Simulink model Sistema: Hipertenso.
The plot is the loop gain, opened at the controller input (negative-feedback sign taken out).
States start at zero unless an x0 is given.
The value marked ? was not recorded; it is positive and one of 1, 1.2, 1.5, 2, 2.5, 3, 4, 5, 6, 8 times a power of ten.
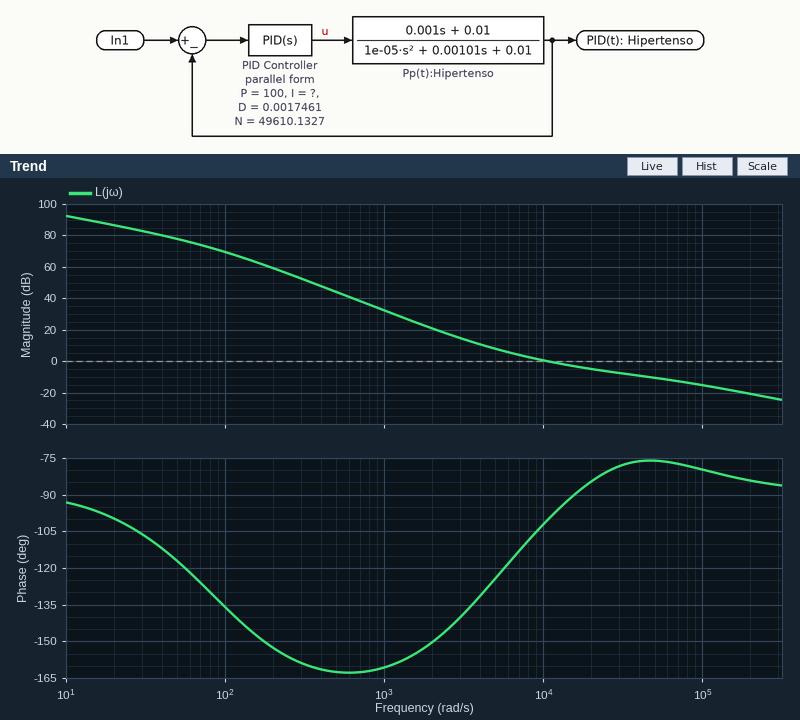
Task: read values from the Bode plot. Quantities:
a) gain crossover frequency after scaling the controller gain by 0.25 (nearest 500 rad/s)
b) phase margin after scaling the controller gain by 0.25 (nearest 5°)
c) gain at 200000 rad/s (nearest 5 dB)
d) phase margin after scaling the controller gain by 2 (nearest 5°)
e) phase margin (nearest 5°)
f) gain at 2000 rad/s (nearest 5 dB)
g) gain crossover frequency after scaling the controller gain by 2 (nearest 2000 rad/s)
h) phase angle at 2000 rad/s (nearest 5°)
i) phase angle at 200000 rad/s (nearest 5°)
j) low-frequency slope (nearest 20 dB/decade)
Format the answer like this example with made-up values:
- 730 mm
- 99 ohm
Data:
- 3500 rad/s
- 45°
- -20 dB
- 100°
- 80°
- 20 dB
- 24000 rad/s
- -150°
- -85°
- -20 dB/decade
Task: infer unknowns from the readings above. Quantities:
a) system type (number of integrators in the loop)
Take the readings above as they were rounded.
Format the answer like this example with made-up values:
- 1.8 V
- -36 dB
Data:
- 1
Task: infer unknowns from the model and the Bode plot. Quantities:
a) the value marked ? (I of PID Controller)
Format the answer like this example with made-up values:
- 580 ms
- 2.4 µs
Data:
- 400000
